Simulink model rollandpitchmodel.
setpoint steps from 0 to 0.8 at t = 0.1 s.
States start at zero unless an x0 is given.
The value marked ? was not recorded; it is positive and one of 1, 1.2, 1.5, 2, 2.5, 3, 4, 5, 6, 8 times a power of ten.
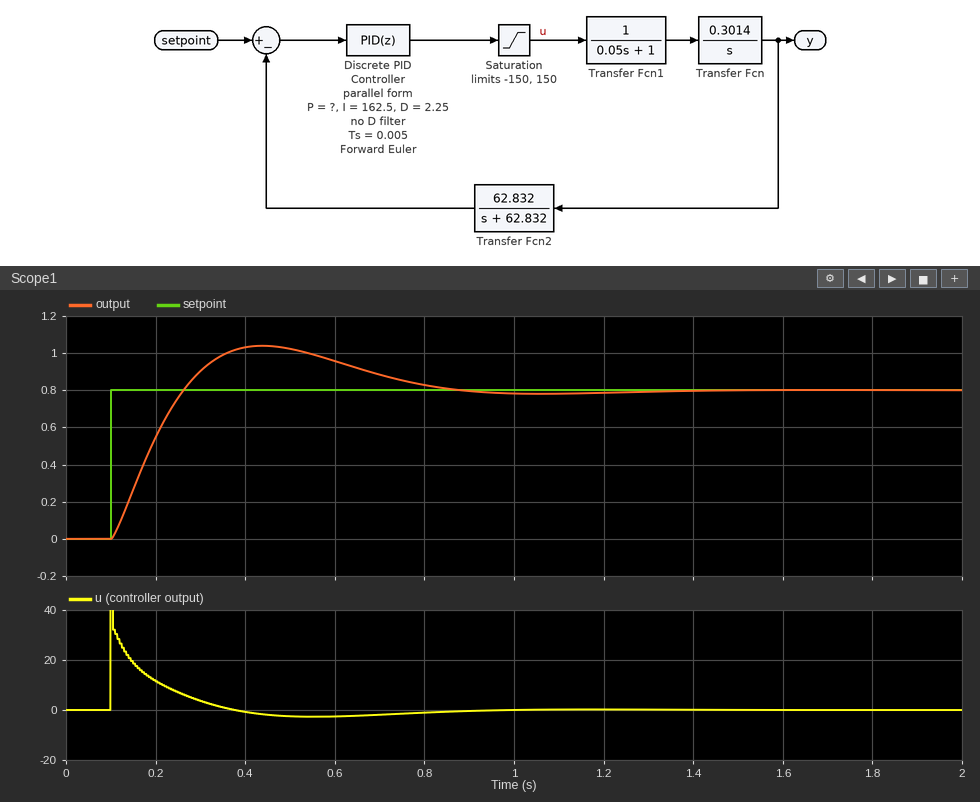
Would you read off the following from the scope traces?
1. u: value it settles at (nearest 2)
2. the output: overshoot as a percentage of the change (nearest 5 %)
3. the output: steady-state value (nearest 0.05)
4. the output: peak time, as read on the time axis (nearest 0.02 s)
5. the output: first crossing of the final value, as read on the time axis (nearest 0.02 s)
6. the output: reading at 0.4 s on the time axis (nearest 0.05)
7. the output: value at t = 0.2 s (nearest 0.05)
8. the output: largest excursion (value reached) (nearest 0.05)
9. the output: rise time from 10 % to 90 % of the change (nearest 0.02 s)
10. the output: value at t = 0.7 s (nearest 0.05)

0
30 %
0.80
0.44 s
0.26 s
1.05
0.55
1.05
0.12 s
0.90
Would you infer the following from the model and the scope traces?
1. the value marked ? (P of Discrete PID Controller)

40
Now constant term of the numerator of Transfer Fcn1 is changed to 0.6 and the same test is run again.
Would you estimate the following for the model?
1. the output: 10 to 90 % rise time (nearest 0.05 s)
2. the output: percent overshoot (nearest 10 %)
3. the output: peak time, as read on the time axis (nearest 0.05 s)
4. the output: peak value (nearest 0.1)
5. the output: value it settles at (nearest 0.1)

0.15 s
40 %
0.55 s
1.1
0.8
